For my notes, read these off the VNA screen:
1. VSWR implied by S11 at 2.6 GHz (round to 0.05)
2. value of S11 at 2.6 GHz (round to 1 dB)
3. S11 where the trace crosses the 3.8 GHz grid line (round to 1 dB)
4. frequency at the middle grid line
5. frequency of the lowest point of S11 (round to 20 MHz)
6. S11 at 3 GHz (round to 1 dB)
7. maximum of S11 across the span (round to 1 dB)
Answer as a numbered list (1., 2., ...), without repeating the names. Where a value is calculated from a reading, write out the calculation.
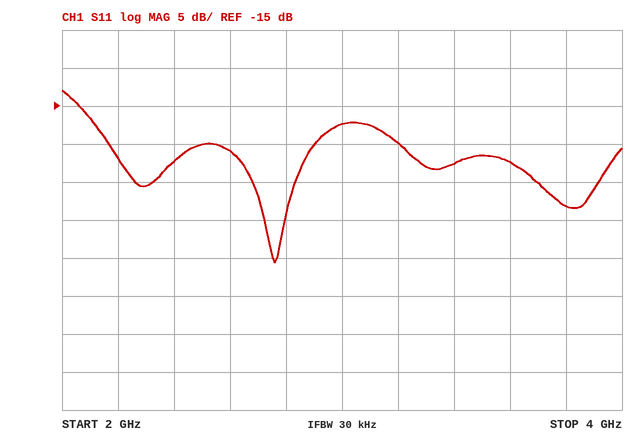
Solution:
1. |Γ| = 10^(-21/20) = 0.0891; VSWR = (1 + 0.0891)/(1 − 0.0891) ≈ 1.20
2. -21 dB
3. -28 dB
4. 3 GHz
5. 2.76 GHz
6. -17 dB
7. -13 dB
